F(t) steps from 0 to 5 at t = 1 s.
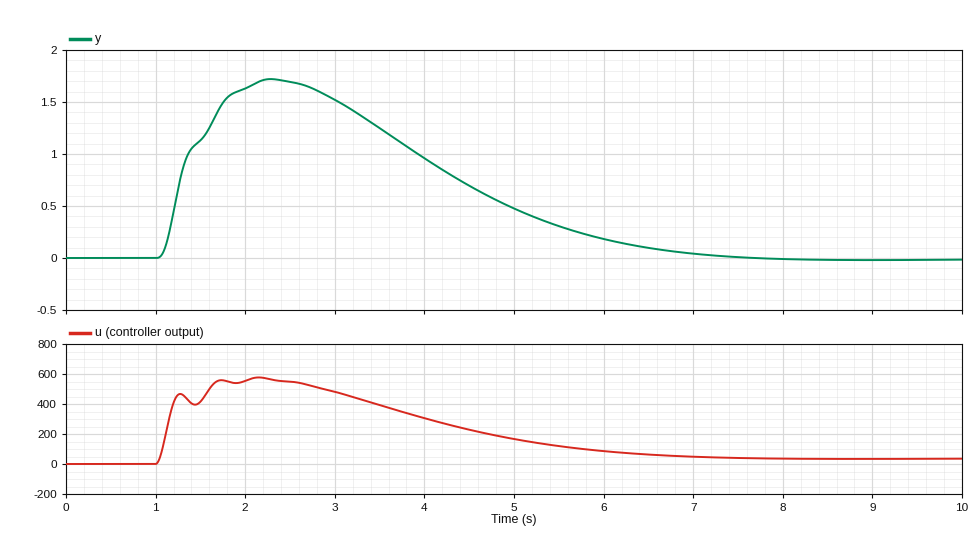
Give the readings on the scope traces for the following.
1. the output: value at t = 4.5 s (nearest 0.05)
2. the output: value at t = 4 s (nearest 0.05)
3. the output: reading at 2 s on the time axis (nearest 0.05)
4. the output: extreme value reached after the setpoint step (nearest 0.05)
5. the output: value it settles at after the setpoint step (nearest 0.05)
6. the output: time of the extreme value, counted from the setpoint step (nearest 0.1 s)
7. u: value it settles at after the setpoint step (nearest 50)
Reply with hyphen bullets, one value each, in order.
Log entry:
- 0.70
- 0.95
- 1.65
- 1.70
- 0.00
- 1.3 s
- 50
